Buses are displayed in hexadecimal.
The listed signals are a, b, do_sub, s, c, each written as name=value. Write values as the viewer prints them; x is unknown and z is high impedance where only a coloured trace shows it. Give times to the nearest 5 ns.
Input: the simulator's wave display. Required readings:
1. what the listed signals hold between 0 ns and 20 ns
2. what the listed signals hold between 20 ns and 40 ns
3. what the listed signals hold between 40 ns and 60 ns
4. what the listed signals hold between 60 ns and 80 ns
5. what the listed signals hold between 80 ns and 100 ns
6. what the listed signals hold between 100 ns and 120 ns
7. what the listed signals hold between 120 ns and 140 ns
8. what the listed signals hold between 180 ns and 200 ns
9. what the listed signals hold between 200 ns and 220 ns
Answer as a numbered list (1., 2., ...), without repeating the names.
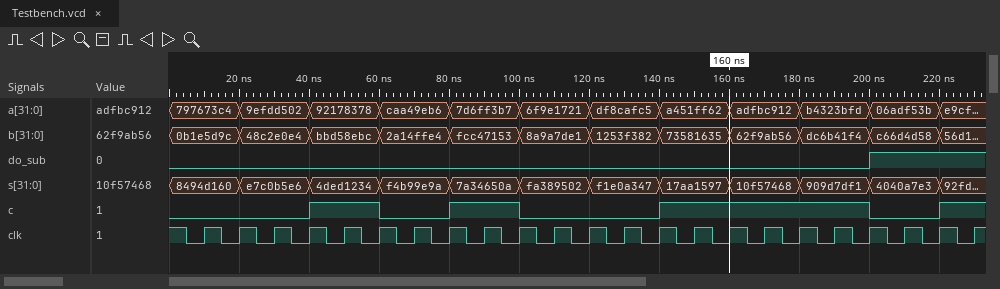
1. a=797673c4, b=0b1e5d9c, do_sub=0, s=8494d160, c=0
2. a=9efdd502, b=48c2e0e4, do_sub=0, s=e7c0b5e6, c=0
3. a=92178378, b=bbd58ebc, do_sub=0, s=4ded1234, c=1
4. a=caa49eb6, b=2a14ffe4, do_sub=0, s=f4b99e9a, c=0
5. a=7d6ff3b7, b=fcc47153, do_sub=0, s=7a34650a, c=1
6. a=6f9e1721, b=8a9a7de1, do_sub=0, s=fa389502, c=0
7. a=df8cafc5, b=1253f382, do_sub=0, s=f1e0a347, c=0
8. a=b4323bfd, b=dc6b41f4, do_sub=0, s=909d7df1, c=1
9. a=06adf53b, b=c66d4d58, do_sub=1, s=4040a7e3, c=0
